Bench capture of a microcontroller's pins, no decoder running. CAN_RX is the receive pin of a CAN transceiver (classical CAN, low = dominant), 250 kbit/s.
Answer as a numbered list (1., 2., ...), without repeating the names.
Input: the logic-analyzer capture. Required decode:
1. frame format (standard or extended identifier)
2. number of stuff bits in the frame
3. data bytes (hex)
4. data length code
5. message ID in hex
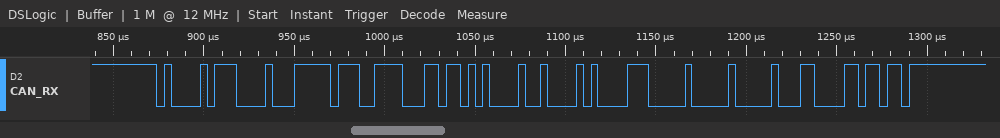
1. standard
2. 4
3. FF 3C 6D 42 42 87 00 00
4. 8
5. 0x42E
